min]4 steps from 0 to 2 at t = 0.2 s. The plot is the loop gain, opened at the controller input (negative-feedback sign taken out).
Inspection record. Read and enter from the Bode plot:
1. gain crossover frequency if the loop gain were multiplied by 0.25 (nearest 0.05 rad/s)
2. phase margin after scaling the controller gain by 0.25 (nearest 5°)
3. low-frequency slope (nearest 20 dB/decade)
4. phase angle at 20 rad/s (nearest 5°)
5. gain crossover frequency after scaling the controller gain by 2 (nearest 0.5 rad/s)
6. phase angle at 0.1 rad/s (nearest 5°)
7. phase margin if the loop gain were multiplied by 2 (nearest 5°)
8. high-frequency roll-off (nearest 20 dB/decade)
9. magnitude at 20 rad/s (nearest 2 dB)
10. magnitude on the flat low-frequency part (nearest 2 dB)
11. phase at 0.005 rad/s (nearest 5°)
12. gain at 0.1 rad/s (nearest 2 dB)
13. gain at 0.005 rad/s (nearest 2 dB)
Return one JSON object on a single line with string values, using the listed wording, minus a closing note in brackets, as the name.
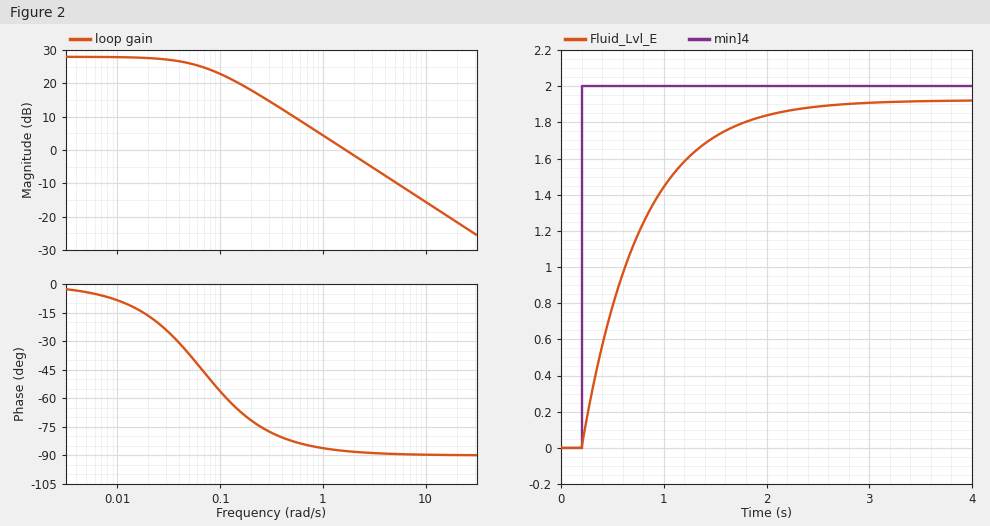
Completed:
{"gain crossover frequency if the loop gain were multiplied by 0.25": "0.40 rad/s", "phase margin after scaling the controller gain by 0.25": "100°", "low-frequency slope": "0 dB/decade", "phase angle at 20 rad/s": "-90°", "gain crossover frequency after scaling the controller gain by 2": "3.5 rad/s", "phase angle at 0.1 rad/s": "-55°", "phase margin if the loop gain were multiplied by 2": "90°", "high-frequency roll-off": "-20 dB/decade", "magnitude at 20 rad/s": "-22 dB", "magnitude on the flat low-frequency part": "28 dB", "phase at 0.005 rad/s": "-5°", "gain at 0.1 rad/s": "22 dB", "gain at 0.005 rad/s": "28 dB"}
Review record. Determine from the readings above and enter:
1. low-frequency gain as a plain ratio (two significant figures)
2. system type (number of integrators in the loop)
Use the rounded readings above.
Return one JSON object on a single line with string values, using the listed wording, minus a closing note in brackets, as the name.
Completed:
{"low-frequency gain as a plain ratio": "25", "system type": "0"}
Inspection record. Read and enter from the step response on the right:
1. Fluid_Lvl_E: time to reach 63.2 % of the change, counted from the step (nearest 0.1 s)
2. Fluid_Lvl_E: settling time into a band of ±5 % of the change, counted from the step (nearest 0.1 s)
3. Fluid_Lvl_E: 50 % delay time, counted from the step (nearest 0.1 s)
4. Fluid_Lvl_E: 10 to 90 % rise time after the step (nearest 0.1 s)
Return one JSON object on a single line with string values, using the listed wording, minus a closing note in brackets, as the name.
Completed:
{"Fluid_Lvl_E: time to reach 63.2 % of the change, counted from the step": "0.6 s", "Fluid_Lvl_E: settling time into a band of ±5 % of the change, counted from the step": "1.7 s", "Fluid_Lvl_E: 50 % delay time, counted from the step": "0.4 s", "Fluid_Lvl_E: 10 to 90 % rise time after the step": "1.3 s"}
